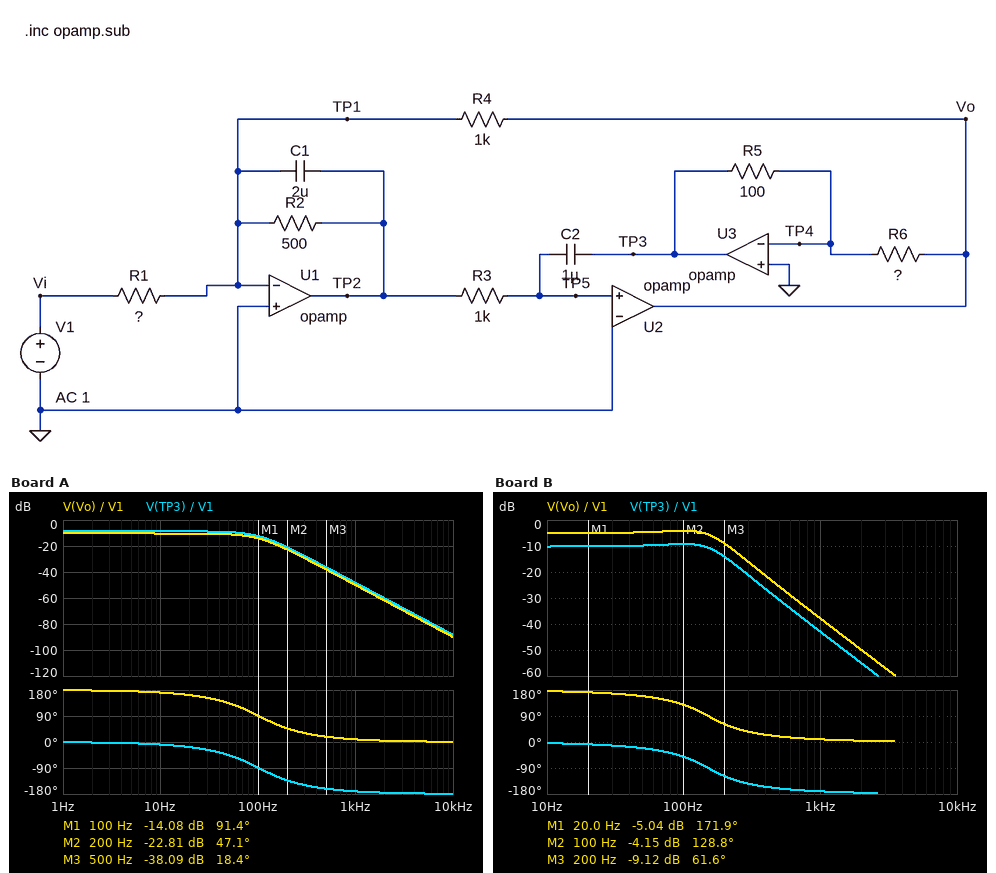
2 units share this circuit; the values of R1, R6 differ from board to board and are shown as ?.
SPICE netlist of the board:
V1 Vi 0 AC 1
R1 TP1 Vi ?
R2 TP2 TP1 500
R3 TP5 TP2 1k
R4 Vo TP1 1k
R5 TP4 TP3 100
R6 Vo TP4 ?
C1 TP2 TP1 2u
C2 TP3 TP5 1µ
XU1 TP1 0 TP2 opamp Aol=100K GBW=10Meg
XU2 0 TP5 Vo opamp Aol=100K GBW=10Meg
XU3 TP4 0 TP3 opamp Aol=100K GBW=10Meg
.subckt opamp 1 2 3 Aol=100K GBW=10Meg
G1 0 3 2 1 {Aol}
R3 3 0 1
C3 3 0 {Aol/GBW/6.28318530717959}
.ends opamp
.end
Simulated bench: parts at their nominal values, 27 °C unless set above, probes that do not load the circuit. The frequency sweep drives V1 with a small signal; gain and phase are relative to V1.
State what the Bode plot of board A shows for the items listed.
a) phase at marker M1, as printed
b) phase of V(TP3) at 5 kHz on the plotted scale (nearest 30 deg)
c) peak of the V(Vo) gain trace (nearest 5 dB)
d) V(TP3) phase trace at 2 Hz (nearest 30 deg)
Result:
91.4 deg
-180 deg
-10 dB
0 deg
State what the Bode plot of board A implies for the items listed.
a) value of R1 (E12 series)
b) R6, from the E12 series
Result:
3.3 kΩ
82 Ω
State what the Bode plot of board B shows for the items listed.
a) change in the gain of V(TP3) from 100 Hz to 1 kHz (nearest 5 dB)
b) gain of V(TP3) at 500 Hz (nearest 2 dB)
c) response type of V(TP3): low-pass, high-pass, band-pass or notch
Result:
-35 dB
-30 dB
low-pass
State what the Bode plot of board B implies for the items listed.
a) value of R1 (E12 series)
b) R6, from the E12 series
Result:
1.8 kΩ
180 Ω
